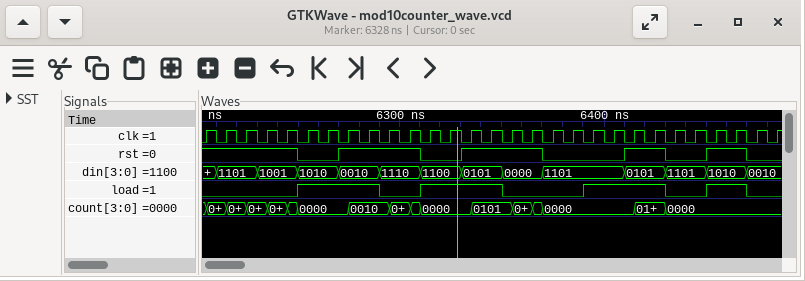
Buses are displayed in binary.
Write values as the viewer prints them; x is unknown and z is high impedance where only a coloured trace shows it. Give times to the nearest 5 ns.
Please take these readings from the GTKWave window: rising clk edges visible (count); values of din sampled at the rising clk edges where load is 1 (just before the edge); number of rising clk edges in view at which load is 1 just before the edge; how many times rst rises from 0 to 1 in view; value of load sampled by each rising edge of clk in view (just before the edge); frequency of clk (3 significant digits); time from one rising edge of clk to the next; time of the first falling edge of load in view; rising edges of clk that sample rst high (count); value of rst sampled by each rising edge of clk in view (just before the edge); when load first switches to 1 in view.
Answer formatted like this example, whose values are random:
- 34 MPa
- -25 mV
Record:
- 29
- 1010, 1010, 0010, 0010, 1100, 1100, 0101, 0101, 1101, 1101, 0101, 0101, 1010, 1010
- 14
- 4
- 0 0 0 0 0 1 1 1 1 0 0 1 1 1 1 0 0 0 0 1 1 1 1 0 0 1 1 0 0
- 100 MHz
- 10 ns
- 6290 ns
- 17
- 1 1 1 1 1 0 0 1 1 1 1 0 0 1 1 1 1 0 0 0 0 1 1 0 0 1 1 0 0
- 6250 ns
